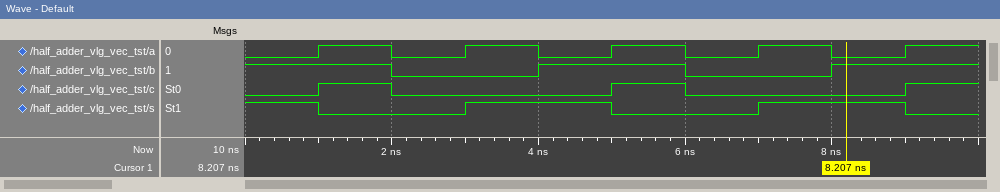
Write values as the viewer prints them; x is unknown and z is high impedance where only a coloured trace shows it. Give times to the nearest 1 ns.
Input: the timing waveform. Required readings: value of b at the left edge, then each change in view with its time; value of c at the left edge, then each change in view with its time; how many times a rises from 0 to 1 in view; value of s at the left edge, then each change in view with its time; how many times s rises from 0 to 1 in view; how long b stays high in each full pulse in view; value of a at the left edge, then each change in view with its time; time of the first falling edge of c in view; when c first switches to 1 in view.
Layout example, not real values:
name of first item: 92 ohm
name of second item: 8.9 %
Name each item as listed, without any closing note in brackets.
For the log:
value of b at the left edge, then each change in view with its time: 1, 0 at 2 ns, 1 at 4 ns, 0 at 6 ns, 1 at 8 ns
value of c at the left edge, then each change in view with its time: 0, 1 at 1 ns, 0 at 2 ns, 1 at 5 ns, 0 at 6 ns, 1 at 9 ns
how many times a rises from 0 to 1 in view: 5
value of s at the left edge, then each change in view with its time: 1, 0 at 1 ns, 1 at 3 ns, 0 at 5 ns, 1 at 7 ns, 0 at 9 ns
how many times s rises from 0 to 1 in view: 2
how long b stays high in each full pulse in view: 2 ns
value of a at the left edge, then each change in view with its time: 0, 1 at 1 ns, 0 at 2 ns, 1 at 3 ns, 0 at 4 ns, 1 at 5 ns, 0 at 6 ns, 1 at 7 ns, 0 at 8 ns, 1 at 9 ns
time of the first falling edge of c in view: 2 ns
when c first switches to 1 in view: 1 ns
